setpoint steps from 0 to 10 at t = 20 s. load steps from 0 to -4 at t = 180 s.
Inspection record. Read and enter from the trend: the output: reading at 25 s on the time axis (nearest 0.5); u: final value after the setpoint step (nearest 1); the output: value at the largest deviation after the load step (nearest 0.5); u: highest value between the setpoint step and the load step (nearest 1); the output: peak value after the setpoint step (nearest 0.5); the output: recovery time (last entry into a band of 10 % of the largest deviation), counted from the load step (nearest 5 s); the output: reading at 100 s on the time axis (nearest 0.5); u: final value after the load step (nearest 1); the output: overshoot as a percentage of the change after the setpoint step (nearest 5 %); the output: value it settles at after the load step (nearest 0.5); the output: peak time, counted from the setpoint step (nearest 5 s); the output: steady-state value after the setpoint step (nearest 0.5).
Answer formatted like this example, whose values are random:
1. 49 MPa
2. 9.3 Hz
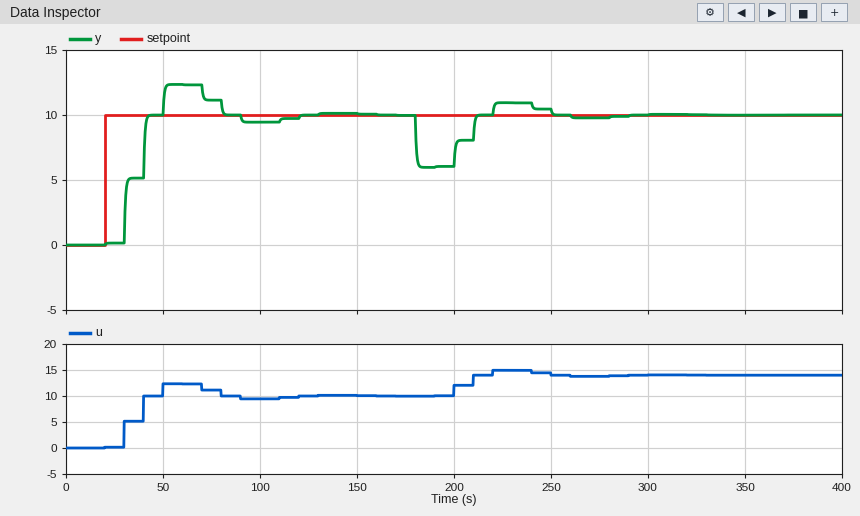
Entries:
1. 0.0
2. 10
3. 6.0
4. 12
5. 12.5
6. 70 s
7. 9.5
8. 14
9. 25 %
10. 10.0
11. 40 s
12. 10.0
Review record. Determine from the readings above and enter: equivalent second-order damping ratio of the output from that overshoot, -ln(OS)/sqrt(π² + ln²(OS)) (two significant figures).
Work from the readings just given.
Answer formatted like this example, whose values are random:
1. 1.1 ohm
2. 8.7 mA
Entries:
1. 0.40
